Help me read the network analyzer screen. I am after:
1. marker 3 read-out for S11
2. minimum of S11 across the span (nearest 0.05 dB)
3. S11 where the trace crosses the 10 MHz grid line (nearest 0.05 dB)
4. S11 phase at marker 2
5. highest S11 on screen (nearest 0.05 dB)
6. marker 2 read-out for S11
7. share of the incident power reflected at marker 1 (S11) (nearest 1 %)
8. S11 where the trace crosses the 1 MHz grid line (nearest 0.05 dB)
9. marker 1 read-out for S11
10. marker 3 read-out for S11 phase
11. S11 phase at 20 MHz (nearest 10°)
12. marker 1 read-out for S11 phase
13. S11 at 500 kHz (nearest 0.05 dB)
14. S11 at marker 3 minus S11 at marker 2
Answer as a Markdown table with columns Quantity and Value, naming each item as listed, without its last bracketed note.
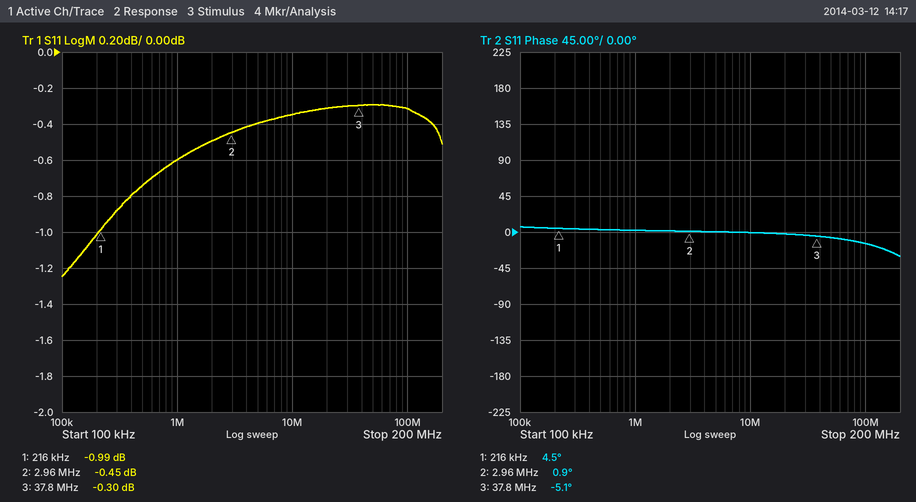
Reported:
| Quantity | Value |
|---|---|
| marker 3 read-out for S11 | -0.30 dB |
| minimum of S11 across the span | -1.25 dB |
| S11 where the trace crosses the 10 MHz grid line | -0.35 dB |
| S11 phase at marker 2 | 0.9° |
| highest S11 on screen | -0.30 dB |
| marker 2 read-out for S11 | -0.45 dB |
| share of the incident power reflected at marker 1 (S11) | 80 % |
| S11 where the trace crosses the 1 MHz grid line | -0.60 dB |
| marker 1 read-out for S11 | -0.99 dB |
| marker 3 read-out for S11 phase | -5.1° |
| S11 phase at 20 MHz | 0° |
| marker 1 read-out for S11 phase | 4.5° |
| S11 at 500 kHz | -0.75 dB |
| S11 at marker 3 minus S11 at marker 2 | 0.15 dB |
